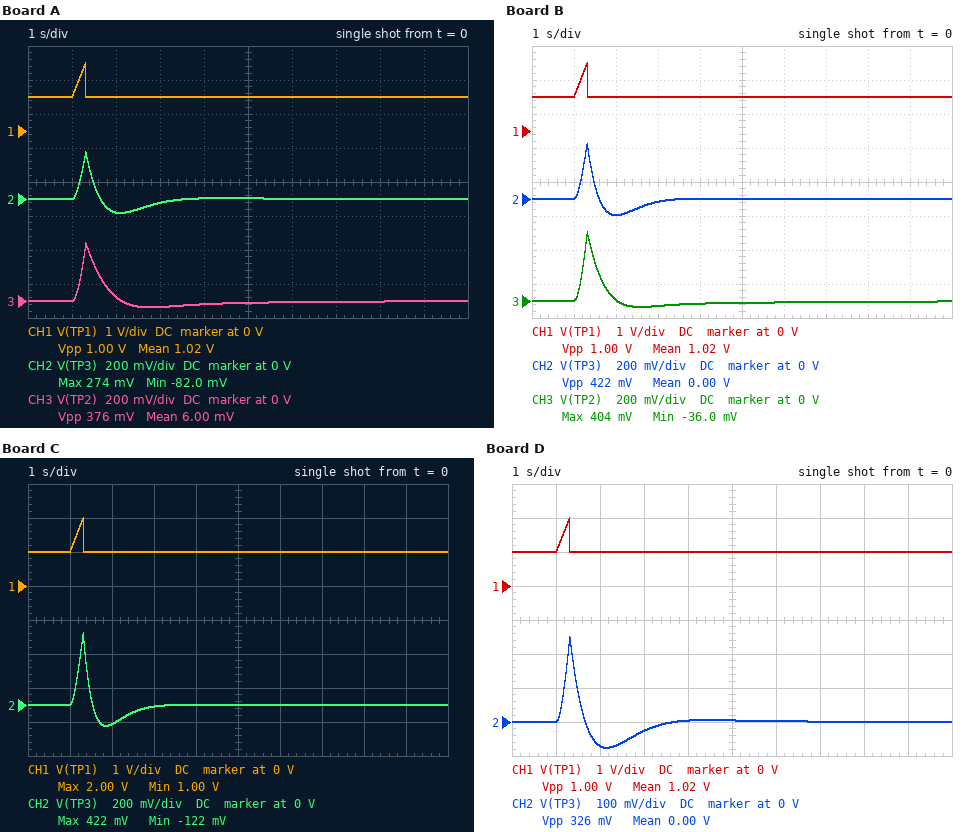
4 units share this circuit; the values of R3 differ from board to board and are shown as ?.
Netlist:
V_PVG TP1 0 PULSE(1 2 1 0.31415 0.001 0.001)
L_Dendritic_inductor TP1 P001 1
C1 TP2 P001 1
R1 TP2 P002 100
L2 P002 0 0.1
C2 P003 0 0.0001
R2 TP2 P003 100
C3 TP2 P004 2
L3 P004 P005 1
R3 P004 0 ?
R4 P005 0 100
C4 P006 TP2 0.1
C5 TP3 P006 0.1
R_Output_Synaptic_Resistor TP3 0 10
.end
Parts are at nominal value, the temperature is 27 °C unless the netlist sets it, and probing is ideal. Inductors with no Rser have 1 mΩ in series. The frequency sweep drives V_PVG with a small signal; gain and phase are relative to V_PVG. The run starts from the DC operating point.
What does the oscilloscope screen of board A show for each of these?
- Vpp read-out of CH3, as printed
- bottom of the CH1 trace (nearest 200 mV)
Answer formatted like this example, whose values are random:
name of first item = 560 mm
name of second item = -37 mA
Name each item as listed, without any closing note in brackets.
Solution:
Vpp read-out of CH3, as printed = 376 mV
bottom of the CH1 trace = 1.0 V
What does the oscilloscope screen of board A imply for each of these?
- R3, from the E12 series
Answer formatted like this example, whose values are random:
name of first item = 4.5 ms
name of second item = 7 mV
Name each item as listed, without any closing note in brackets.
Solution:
R3, from the E12 series = 3.9 Ω
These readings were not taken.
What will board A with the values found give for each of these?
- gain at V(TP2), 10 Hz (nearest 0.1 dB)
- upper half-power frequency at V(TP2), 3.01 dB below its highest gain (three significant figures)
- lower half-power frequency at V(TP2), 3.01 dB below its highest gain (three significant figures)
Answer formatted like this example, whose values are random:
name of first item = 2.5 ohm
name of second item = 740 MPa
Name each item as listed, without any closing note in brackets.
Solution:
gain at V(TP2), 10 Hz = -27.5 dB
upper half-power frequency at V(TP2), 3.01 dB below its highest gain = 545 mHz
lower half-power frequency at V(TP2), 3.01 dB below its highest gain = 58.2 mHz
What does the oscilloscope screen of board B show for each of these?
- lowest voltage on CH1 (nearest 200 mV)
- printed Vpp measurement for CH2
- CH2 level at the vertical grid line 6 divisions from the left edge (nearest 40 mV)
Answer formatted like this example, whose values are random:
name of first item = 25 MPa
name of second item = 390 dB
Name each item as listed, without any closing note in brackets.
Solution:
lowest voltage on CH1 = 1.0 V
printed Vpp measurement for CH2 = 422 mV
CH2 level at the vertical grid line 6 divisions from the left edge = 0 V
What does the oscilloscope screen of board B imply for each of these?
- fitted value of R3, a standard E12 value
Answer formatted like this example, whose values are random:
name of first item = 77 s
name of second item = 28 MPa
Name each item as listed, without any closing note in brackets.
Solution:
fitted value of R3, a standard E12 value = 5.6 Ω
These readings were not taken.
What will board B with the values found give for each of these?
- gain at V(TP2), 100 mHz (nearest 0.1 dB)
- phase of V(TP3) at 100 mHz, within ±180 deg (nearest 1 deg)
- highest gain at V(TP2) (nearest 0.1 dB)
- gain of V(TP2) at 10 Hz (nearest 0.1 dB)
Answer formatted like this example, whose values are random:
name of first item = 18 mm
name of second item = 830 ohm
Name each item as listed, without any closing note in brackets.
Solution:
gain at V(TP2), 100 mHz = -0.6 dB
phase of V(TP3) at 100 mHz, within ±180 deg = 83 deg
highest gain at V(TP2) = 0.3 dB
gain of V(TP2) at 10 Hz = -25.5 dB
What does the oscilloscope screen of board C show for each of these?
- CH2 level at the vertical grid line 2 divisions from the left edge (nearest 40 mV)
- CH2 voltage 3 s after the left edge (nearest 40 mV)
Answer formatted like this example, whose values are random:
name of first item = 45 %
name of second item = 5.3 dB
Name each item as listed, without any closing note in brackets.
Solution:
CH2 level at the vertical grid line 2 divisions from the left edge = -120 mV
CH2 voltage 3 s after the left edge = 0 V
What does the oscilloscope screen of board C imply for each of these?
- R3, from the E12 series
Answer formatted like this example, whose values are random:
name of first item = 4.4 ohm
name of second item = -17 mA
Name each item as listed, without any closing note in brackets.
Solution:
R3, from the E12 series = 12 Ω
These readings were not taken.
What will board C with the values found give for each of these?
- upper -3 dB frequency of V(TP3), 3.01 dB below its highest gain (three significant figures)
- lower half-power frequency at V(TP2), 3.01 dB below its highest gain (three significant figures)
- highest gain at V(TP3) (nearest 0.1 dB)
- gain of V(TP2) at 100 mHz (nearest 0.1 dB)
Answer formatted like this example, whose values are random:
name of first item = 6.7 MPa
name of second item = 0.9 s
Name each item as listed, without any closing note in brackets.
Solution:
upper -3 dB frequency of V(TP3), 3.01 dB below its highest gain = 1.15 Hz
lower half-power frequency at V(TP2), 3.01 dB below its highest gain = 25.2 mHz
highest gain at V(TP3) = -1.5 dB
gain of V(TP2) at 100 mHz = -0.3 dB
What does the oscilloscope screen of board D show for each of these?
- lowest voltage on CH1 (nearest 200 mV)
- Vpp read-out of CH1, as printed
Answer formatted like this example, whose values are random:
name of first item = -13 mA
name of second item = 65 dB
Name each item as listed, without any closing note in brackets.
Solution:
lowest voltage on CH1 = 1.0 V
Vpp read-out of CH1, as printed = 1.00 V
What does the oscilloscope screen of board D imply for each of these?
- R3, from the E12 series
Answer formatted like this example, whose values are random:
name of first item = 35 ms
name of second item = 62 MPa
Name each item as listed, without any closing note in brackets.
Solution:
R3, from the E12 series = 3.3 Ω
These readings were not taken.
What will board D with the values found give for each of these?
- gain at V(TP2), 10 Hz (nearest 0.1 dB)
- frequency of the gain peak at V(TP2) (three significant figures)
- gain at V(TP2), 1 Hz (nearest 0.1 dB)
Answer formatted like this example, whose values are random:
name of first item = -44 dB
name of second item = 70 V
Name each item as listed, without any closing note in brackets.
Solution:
gain at V(TP2), 10 Hz = -28.5 dB
frequency of the gain peak at V(TP2) = 212 mHz
gain at V(TP2), 1 Hz = -8.5 dB
